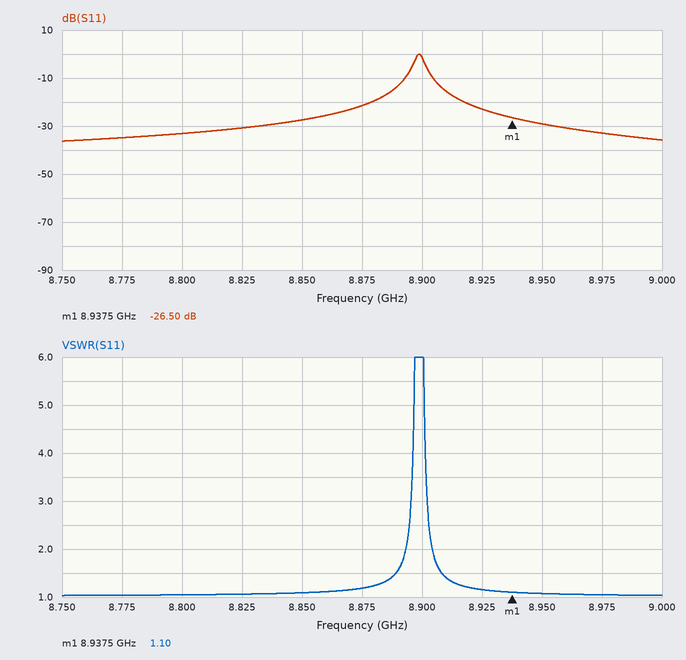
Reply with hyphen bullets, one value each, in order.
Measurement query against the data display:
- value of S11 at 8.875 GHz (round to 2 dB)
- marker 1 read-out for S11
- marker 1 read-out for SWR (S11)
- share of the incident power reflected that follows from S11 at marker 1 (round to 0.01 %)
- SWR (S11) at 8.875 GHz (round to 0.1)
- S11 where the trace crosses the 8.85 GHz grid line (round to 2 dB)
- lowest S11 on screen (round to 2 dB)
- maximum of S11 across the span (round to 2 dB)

- -22 dB
- -26.50 dB
- 1.10
- 0.22 %
- 1.2
- -28 dB
- -36 dB
- 0 dB
